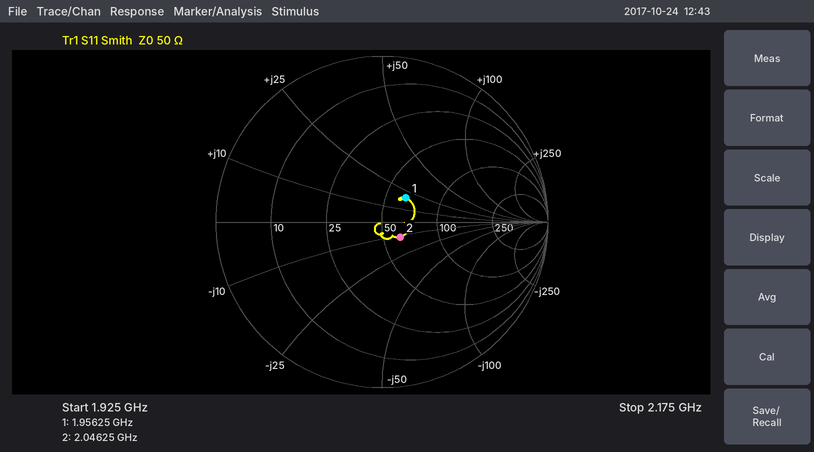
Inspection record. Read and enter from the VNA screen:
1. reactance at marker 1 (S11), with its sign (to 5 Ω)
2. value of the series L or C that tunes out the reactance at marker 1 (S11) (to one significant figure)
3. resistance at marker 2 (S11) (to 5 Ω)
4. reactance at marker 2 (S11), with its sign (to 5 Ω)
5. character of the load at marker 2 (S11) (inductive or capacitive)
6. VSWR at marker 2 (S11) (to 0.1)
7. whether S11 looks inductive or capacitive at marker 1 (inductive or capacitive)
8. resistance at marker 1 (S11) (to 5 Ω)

+20 Ω
4 pF
60 Ω
-10 Ω
capacitive
1.3
inductive
65 Ω
